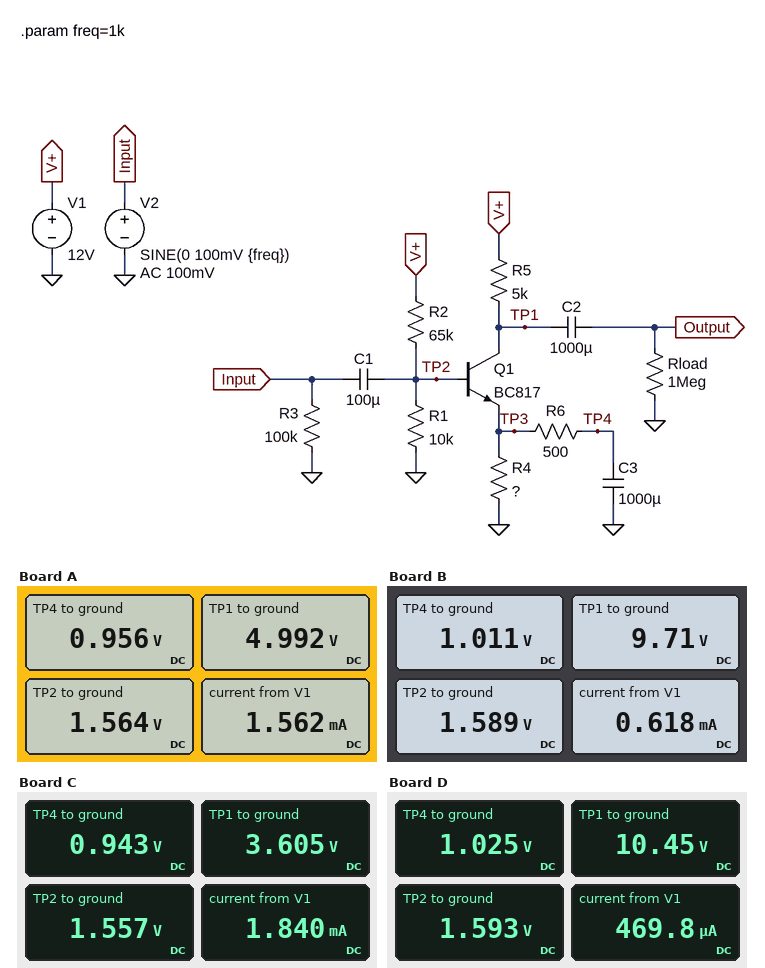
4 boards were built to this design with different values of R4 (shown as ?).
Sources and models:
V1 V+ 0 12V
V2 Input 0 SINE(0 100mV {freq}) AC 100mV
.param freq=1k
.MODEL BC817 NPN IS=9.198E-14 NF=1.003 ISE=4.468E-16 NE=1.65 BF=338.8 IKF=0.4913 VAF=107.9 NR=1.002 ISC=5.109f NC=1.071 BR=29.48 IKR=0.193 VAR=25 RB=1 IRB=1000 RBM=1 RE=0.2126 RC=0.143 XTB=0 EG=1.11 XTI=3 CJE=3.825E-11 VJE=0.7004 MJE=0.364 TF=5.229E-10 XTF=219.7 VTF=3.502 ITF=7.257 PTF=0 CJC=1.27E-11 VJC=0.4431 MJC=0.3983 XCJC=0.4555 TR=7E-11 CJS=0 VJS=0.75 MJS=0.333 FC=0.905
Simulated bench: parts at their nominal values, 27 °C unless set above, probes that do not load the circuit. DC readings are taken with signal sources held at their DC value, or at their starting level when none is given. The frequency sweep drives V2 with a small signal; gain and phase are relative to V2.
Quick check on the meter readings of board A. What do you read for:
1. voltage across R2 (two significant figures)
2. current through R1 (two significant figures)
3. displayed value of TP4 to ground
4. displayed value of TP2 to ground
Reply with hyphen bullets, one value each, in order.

- 10 V
- 160 µA
- 0.956 V
- 1.564 V
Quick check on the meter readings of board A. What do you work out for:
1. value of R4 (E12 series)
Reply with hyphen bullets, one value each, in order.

- 680 Ω
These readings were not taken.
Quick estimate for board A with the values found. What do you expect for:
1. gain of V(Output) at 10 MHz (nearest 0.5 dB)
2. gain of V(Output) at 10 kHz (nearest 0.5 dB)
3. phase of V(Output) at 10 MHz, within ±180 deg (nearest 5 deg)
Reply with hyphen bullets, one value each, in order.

- 18.5 dB
- 24.0 dB
- 110 deg
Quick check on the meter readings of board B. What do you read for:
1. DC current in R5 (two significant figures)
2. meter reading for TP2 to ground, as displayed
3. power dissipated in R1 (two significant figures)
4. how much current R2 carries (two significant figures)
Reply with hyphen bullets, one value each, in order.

- 460 µA
- 1.589 V
- 250 µW
- 160 µA
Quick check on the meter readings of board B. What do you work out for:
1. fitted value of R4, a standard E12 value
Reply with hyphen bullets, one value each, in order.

- 2.2 kΩ
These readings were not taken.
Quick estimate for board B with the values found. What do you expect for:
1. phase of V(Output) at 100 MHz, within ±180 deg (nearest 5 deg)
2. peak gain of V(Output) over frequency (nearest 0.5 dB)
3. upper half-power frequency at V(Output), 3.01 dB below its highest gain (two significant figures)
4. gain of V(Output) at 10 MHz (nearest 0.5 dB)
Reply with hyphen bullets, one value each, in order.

- 10 deg
- 20.5 dB
- 8.2 MHz
- 16.5 dB
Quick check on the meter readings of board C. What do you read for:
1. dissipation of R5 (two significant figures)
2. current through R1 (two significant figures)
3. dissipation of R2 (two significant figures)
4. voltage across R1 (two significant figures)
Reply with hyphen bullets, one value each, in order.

- 14 mW
- 160 µA
- 1.7 mW
- 1.6 V
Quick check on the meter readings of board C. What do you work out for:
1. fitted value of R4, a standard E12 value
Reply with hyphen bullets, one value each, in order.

- 560 Ω
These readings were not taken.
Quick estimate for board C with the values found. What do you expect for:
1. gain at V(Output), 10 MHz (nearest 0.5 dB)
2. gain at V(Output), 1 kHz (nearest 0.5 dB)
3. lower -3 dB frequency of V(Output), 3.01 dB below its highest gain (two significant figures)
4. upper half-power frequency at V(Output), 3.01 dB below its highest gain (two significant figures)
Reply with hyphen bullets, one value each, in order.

- 18.0 dB
- 25.0 dB
- 350 mHz
- 5.0 MHz
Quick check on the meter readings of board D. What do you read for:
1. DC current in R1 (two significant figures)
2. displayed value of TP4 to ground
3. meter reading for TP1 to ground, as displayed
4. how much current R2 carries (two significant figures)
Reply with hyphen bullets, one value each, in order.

- 160 µA
- 1.025 V
- 10.45 V
- 160 µA
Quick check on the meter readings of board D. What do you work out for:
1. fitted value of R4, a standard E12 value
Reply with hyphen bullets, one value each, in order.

- 3.3 kΩ
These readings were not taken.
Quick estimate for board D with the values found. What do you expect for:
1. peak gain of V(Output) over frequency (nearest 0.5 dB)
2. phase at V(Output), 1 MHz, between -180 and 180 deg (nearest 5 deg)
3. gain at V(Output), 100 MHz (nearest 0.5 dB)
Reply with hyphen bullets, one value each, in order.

- 19.5 dB
- 170 deg
- 1.5 dB
